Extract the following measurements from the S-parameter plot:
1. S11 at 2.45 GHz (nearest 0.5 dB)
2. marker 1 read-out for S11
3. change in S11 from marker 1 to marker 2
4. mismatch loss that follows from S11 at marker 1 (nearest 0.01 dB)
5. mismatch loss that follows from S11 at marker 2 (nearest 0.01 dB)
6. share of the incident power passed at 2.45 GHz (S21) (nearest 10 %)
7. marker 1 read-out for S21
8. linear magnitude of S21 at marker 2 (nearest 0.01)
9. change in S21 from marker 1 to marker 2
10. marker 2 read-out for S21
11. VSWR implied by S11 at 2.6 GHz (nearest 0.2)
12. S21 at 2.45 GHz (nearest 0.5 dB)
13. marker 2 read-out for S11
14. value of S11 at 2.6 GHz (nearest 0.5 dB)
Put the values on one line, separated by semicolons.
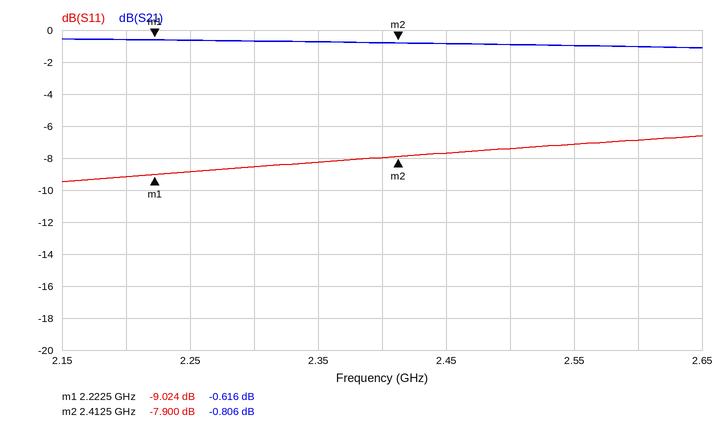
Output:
-7.5 dB; -9.024 dB; 1.124 dB; 0.58 dB; 0.77 dB; 80 %; -0.616 dB; 0.91; -0.190 dB; -0.806 dB; 2.6; -1.0 dB; -7.900 dB; -7.0 dB
